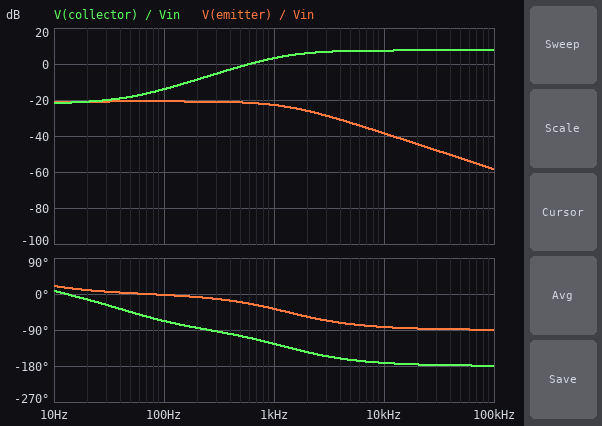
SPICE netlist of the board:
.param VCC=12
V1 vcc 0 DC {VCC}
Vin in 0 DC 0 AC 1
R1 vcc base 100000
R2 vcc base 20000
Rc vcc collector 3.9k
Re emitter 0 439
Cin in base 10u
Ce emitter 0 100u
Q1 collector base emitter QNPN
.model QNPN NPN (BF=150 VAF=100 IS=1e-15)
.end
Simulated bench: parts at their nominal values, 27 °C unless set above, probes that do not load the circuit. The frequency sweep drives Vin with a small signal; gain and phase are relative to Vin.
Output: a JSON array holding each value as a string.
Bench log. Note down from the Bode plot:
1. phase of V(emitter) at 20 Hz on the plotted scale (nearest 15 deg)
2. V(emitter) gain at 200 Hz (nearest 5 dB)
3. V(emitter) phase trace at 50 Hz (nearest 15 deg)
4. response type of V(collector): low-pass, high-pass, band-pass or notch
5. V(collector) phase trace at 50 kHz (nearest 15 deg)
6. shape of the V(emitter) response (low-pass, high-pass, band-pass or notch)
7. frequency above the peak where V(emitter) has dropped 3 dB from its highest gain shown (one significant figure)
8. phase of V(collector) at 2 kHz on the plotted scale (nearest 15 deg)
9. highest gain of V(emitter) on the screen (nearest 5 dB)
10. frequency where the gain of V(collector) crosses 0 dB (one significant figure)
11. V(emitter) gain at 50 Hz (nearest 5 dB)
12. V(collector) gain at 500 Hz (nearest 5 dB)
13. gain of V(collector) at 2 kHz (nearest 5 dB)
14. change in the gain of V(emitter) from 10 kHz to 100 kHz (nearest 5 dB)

["15 deg", "-20 dB", "0 deg", "high-pass", "-180 deg", "low-pass", "1 kHz", "-150 deg", "-20 dB", "600 Hz", "-20 dB", "0 dB", "5 dB", "-20 dB"]
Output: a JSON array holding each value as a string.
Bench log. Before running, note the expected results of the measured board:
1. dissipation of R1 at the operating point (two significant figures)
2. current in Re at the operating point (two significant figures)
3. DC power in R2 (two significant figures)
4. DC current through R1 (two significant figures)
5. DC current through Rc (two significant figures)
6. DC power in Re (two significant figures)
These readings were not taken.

["960 µW", "3.3 mA", "4.8 mW", "98 µA", "2.7 mA", "4.7 mW"]
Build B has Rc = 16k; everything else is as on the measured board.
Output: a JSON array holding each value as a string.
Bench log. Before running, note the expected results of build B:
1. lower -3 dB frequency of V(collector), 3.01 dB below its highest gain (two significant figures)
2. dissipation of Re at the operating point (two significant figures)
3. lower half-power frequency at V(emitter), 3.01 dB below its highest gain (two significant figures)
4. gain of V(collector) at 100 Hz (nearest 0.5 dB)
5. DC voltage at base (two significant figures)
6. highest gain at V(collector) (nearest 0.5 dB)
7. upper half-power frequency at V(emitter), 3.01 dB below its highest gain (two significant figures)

["660 Hz", "800 µW", "3.4 Hz", "-18.5 dB", "1.3 V", "-5.0 dB", "680 Hz"]
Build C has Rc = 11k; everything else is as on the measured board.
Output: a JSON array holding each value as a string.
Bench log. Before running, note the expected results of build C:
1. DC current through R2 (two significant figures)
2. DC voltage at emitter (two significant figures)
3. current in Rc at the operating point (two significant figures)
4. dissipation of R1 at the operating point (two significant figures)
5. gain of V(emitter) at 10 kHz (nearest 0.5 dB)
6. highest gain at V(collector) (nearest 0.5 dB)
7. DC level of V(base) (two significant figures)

["530 µA", "730 mV", "1.0 mA", "1.1 mW", "-43.0 dB", "-1.5 dB", "1.5 V"]
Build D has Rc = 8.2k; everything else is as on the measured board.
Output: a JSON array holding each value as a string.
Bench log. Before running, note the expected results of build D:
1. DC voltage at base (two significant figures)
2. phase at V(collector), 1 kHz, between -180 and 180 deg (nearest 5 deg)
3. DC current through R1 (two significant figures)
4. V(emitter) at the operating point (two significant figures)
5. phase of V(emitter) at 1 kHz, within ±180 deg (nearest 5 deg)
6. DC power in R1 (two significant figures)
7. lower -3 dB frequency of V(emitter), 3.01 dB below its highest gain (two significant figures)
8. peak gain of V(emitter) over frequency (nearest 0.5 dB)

["1.6 V", "-135 deg", "100 µA", "870 mV", "-50 deg", "1.1 mW", "3.5 Hz", "-21.0 dB"]
